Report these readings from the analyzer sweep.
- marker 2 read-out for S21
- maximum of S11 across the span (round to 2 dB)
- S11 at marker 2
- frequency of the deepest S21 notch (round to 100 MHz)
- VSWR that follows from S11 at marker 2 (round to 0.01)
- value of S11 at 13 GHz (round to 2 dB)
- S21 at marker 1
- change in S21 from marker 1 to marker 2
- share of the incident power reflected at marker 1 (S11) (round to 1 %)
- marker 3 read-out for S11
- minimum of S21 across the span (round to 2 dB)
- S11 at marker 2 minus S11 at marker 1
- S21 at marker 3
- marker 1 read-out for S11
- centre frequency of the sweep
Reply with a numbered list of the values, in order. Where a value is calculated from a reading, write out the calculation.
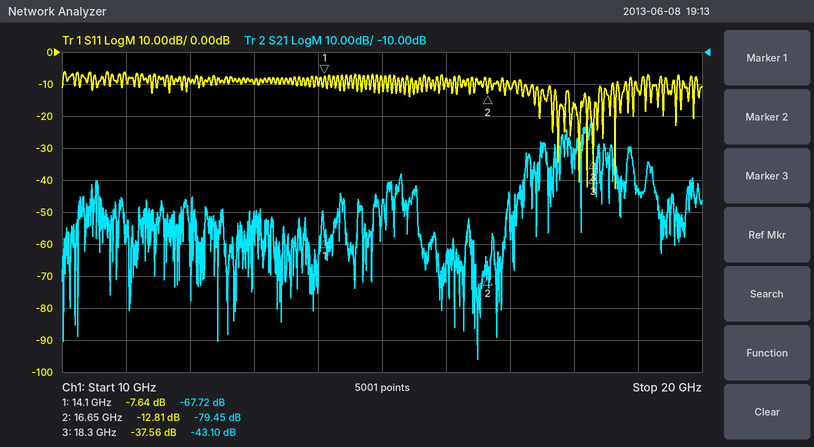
1. -79.45 dB
2. -6 dB
3. -12.81 dB
4. 16.5 GHz
5. (1 + 0.2288)/(1 − 0.2288) ≈ 1.59
6. -10 dB
7. -67.72 dB
8. -79.45 − (-67.72) = -11.73 dB
9. 10^(-7.64/10) ≈ 17 %
10. -37.56 dB
11. -106 dB
12. -12.81 − (-7.64) = -5.17 dB
13. -43.10 dB
14. -7.64 dB
15. 15 GHz
